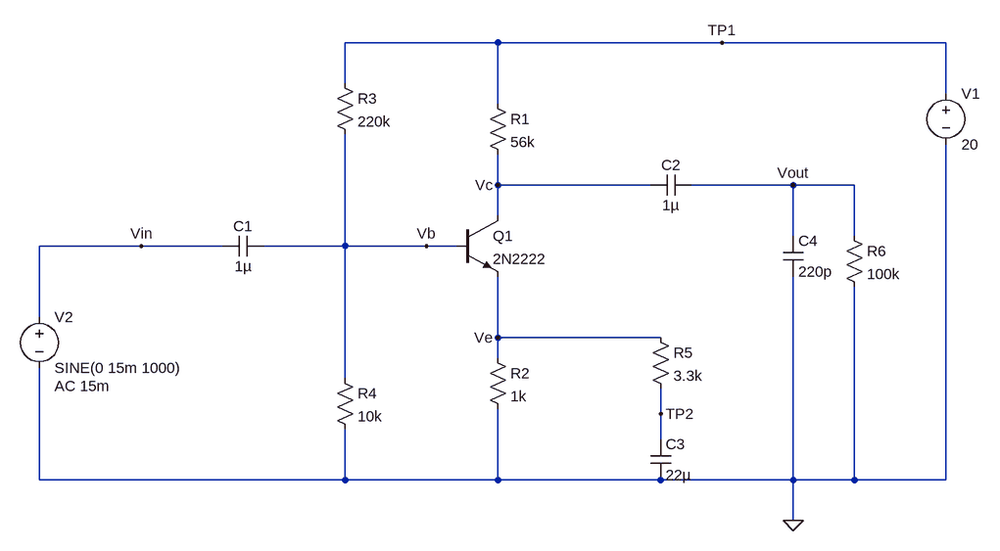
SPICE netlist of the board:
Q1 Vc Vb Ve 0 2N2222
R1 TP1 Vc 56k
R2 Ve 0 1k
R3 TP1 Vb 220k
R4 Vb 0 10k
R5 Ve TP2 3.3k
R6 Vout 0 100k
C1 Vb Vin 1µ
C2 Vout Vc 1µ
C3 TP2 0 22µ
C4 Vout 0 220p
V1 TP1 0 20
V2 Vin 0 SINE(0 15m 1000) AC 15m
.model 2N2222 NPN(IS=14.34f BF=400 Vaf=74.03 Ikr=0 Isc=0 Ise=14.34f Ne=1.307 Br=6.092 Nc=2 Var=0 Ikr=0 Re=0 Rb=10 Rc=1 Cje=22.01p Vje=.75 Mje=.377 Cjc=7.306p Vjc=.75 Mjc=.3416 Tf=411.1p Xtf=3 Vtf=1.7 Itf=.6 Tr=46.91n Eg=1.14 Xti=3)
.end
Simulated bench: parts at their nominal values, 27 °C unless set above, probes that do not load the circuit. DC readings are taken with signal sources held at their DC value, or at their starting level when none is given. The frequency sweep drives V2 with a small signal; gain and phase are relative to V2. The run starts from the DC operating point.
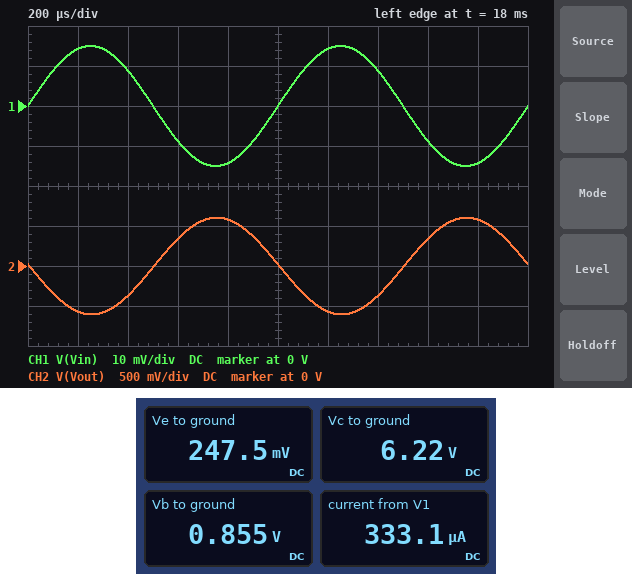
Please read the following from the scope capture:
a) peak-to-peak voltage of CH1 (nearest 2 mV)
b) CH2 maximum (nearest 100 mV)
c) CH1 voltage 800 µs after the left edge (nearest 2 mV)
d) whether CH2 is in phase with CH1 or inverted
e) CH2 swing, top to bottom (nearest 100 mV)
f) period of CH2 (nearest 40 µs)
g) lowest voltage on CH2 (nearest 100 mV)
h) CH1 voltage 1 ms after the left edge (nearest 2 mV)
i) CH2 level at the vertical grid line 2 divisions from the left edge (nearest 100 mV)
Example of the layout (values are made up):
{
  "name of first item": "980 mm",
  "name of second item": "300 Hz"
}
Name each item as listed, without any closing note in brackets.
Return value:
{
  "peak-to-peak voltage of CH1": "30 mV",
  "CH2 maximum": "600 mV",
  "CH1 voltage 800 µs after the left edge": "-14 mV",
  "whether CH2 is in phase with CH1 or inverted": "inverted",
  "CH2 swing, top to bottom": "1.2 V",
  "period of CH2": "1.00 ms",
  "lowest voltage on CH2": "-600 mV",
  "CH1 voltage 1 ms after the left edge": "0 V",
  "CH2 level at the vertical grid line 2 divisions from the left edge": "-400 mV"
}
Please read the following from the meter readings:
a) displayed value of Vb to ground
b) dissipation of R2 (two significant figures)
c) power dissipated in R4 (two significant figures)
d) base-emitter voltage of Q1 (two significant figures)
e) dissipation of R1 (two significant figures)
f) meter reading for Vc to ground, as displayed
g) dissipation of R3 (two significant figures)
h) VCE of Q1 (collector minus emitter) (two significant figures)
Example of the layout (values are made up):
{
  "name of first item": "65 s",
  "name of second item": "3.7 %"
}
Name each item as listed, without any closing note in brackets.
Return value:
{
  "displayed value of Vb to ground": "0.855 V",
  "dissipation of R2": "61 µW",
  "power dissipated in R4": "73 µW",
  "base-emitter voltage of Q1": "610 mV",
  "dissipation of R1": "3.4 mW",
  "meter reading for Vc to ground, as displayed": "6.22 V",
  "dissipation of R3": "1.7 mW",
  "VCE of Q1 (collector minus emitter)": "6.0 V"
}
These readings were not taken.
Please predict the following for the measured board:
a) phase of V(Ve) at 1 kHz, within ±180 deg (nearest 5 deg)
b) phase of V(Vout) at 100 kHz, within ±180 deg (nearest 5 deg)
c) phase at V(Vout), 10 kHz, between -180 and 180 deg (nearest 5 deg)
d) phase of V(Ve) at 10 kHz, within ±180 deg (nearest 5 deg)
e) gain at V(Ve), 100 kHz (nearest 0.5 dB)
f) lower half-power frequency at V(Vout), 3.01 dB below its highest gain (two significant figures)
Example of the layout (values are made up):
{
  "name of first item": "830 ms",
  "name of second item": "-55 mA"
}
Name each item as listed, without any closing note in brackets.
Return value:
{
  "phase of V(Ve) at 1 kHz, within ±180 deg": "0 deg",
  "phase of V(Vout) at 100 kHz, within ±180 deg": "100 deg",
  "phase at V(Vout), 10 kHz, between -180 and 180 deg": "155 deg",
  "phase of V(Ve) at 10 kHz, within ±180 deg": "0 deg",
  "gain at V(Ve), 100 kHz": "-1.0 dB",
  "lower half-power frequency at V(Vout), 3.01 dB below its highest gain": "18 Hz"
}
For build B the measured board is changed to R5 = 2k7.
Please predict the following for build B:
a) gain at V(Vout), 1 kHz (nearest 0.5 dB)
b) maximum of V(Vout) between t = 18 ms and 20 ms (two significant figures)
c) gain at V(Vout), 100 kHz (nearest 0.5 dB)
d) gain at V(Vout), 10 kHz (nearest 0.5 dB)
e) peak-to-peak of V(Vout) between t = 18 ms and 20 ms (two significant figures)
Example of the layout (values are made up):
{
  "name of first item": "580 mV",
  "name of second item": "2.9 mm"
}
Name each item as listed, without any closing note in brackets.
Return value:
{
  "gain at V(Vout), 1 kHz": "32.5 dB",
  "maximum of V(Vout) between t = 18 ms and 20 ms": "630 mV",
  "gain at V(Vout), 100 kHz": "18.5 dB",
  "gain at V(Vout), 10 kHz": "31.5 dB",
  "peak-to-peak of V(Vout) between t = 18 ms and 20 ms": "1.3 V"
}
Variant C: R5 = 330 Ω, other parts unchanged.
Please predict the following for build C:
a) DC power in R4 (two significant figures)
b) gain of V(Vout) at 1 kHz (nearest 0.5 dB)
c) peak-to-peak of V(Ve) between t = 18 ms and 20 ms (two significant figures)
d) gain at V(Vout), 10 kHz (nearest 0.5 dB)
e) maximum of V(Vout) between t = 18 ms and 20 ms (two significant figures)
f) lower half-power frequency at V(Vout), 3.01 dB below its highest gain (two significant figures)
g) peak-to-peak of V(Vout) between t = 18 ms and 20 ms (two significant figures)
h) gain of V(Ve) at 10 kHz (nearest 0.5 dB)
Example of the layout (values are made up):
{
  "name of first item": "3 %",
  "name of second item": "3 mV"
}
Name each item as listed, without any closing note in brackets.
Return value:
{
  "DC power in R4": "73 µW",
  "gain of V(Vout) at 1 kHz": "40.0 dB",
  "peak-to-peak of V(Ve) between t = 18 ms and 20 ms": "20 mV",
  "gain at V(Vout), 10 kHz": "39.0 dB",
  "maximum of V(Vout) between t = 18 ms and 20 ms": "1.4 V",
  "lower half-power frequency at V(Vout), 3.01 dB below its highest gain": "27 Hz",
  "peak-to-peak of V(Vout) between t = 18 ms and 20 ms": "2.9 V",
  "gain of V(Ve) at 10 kHz": "-3.5 dB"
}
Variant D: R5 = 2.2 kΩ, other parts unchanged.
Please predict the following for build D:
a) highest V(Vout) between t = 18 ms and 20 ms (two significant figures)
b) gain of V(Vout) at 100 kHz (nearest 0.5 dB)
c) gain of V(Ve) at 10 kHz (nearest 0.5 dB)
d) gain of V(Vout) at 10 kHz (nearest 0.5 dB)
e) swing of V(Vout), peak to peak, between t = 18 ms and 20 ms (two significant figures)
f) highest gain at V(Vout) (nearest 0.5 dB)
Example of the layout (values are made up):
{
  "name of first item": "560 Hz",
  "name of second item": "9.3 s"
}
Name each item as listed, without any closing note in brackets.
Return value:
{
  "highest V(Vout) between t = 18 ms and 20 ms": "660 mV",
  "gain of V(Vout) at 100 kHz": "19.0 dB",
  "gain of V(Ve) at 10 kHz": "-1.5 dB",
  "gain of V(Vout) at 10 kHz": "32.0 dB",
  "swing of V(Vout), peak to peak, between t = 18 ms and 20 ms": "1.3 V",
  "highest gain at V(Vout)": "33.0 dB"
}
